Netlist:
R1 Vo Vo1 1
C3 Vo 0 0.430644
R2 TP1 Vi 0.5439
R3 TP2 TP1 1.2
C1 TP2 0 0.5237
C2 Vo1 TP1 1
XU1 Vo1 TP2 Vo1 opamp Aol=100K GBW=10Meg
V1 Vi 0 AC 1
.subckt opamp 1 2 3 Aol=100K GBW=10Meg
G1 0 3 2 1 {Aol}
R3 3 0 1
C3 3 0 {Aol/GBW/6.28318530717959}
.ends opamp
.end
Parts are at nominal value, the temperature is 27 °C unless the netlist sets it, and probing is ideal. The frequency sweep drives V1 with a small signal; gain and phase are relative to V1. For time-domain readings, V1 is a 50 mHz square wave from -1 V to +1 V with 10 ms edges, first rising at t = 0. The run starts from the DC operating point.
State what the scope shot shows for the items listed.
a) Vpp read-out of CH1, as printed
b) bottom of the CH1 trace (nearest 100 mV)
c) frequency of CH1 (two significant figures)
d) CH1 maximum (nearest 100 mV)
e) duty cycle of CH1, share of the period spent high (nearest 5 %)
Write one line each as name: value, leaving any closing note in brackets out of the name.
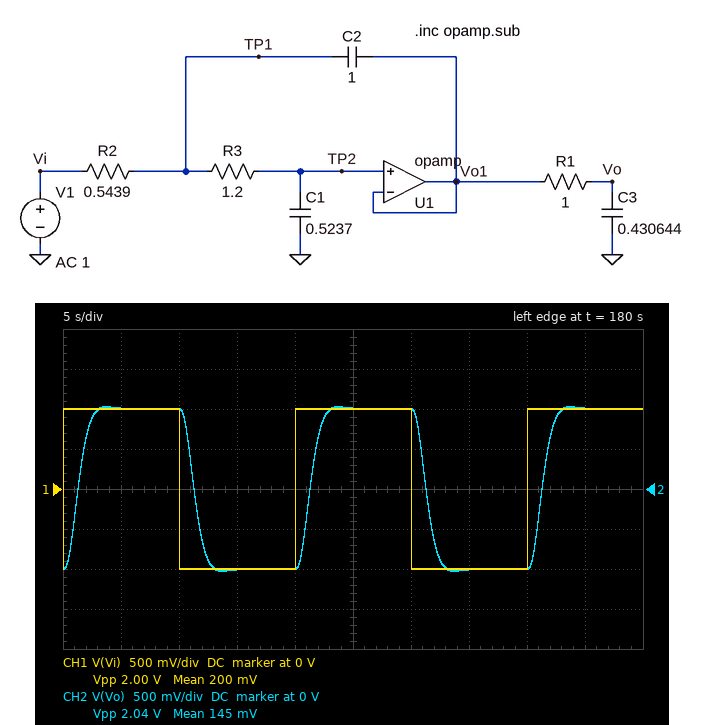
Vpp read-out of CH1, as printed: 2.00 V
bottom of the CH1 trace: -1.0 V
frequency of CH1: 50 mHz
CH1 maximum: 1.0 V
duty cycle of CH1, share of the period spent high: 50 %
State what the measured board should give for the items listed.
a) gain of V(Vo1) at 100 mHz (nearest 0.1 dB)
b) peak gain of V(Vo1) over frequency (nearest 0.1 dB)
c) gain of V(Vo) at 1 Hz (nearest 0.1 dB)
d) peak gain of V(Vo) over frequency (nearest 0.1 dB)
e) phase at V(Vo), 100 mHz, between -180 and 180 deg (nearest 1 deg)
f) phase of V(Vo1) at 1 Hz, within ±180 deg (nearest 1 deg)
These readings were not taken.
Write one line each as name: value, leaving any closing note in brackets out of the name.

gain of V(Vo1) at 100 mHz: -0.3 dB
peak gain of V(Vo1) over frequency: 0 dB
gain of V(Vo) at 1 Hz: -32.0 dB
peak gain of V(Vo) over frequency: 0 dB
phase at V(Vo), 100 mHz, between -180 and 180 deg: -49 deg
phase of V(Vo1) at 1 Hz, within ±180 deg: -155 deg
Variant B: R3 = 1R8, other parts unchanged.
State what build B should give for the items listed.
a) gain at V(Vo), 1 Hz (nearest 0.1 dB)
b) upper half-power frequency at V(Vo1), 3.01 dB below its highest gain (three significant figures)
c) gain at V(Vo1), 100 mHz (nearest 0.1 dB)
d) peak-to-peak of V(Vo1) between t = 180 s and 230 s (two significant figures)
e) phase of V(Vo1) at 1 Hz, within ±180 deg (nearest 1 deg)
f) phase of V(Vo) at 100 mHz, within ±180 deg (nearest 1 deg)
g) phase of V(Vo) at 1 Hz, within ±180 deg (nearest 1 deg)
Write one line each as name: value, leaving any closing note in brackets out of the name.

gain at V(Vo), 1 Hz: -35.5 dB
upper half-power frequency at V(Vo1), 3.01 dB below its highest gain: 177 mHz
gain at V(Vo1), 100 mHz: -0.9 dB
peak-to-peak of V(Vo1) between t = 180 s and 230 s: 2.0 V
phase of V(Vo1) at 1 Hz, within ±180 deg: -158 deg
phase of V(Vo) at 100 mHz, within ±180 deg: -59 deg
phase of V(Vo) at 1 Hz, within ±180 deg: 132 deg
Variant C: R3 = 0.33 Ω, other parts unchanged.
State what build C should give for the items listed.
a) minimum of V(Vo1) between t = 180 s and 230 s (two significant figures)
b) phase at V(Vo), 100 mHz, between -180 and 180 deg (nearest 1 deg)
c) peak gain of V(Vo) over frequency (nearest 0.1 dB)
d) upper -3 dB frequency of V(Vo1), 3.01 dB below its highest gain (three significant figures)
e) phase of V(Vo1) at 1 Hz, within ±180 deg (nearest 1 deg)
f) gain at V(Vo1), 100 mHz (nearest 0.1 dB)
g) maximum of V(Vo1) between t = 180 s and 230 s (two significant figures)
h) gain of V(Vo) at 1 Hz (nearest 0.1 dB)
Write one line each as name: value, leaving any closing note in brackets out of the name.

minimum of V(Vo1) between t = 180 s and 230 s: -1.1 V
phase at V(Vo), 100 mHz, between -180 and 180 deg: -32 deg
peak gain of V(Vo) over frequency: 0 dB
upper -3 dB frequency of V(Vo1), 3.01 dB below its highest gain: 490 mHz
phase of V(Vo1) at 1 Hz, within ±180 deg: -133 deg
gain at V(Vo1), 100 mHz: 0 dB
maximum of V(Vo1) between t = 180 s and 230 s: 1.1 V
gain of V(Vo) at 1 Hz: -21.1 dB
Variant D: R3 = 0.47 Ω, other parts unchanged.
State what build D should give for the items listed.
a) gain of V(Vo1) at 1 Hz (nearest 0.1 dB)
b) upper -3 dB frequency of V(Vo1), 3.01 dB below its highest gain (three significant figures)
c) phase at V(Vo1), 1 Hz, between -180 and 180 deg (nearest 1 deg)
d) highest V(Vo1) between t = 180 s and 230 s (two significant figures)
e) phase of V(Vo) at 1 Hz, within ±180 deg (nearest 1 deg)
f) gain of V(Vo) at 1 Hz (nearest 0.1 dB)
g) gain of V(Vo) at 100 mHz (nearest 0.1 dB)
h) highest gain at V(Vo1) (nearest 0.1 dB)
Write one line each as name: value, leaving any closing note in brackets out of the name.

gain of V(Vo1) at 1 Hz: -14.7 dB
upper -3 dB frequency of V(Vo1), 3.01 dB below its highest gain: 424 mHz
phase at V(Vo1), 1 Hz, between -180 and 180 deg: -142 deg
highest V(Vo1) between t = 180 s and 230 s: 1.1 V
phase of V(Vo) at 1 Hz, within ±180 deg: 148 deg
gain of V(Vo) at 1 Hz: -23.9 dB
gain of V(Vo) at 100 mHz: -0.3 dB
highest gain at V(Vo1): 0 dB
